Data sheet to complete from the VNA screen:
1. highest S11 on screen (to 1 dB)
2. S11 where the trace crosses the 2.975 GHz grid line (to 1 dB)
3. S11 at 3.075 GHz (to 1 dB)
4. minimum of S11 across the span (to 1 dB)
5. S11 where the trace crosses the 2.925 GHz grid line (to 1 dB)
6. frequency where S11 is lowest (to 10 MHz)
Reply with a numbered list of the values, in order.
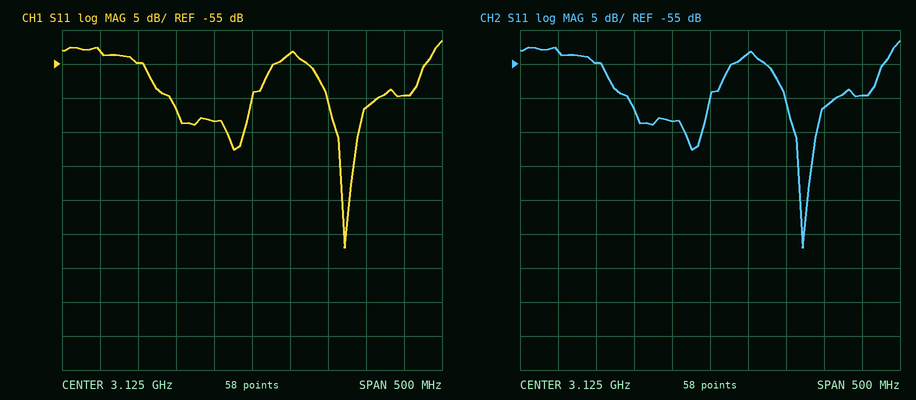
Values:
1. -52 dB
2. -55 dB
3. -63 dB
4. -82 dB
5. -53 dB
6. 3.25 GHz
